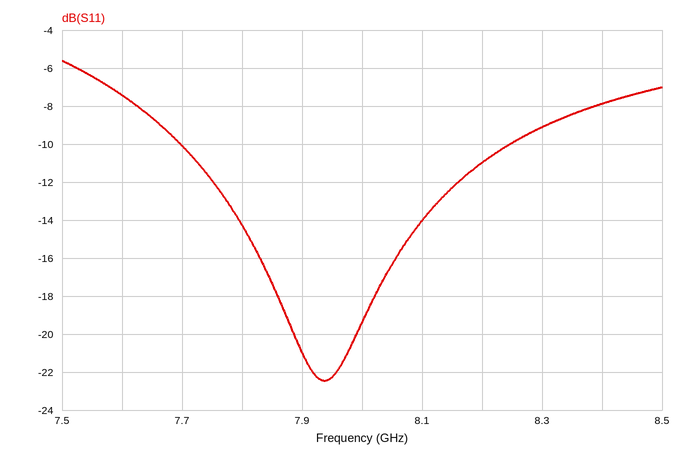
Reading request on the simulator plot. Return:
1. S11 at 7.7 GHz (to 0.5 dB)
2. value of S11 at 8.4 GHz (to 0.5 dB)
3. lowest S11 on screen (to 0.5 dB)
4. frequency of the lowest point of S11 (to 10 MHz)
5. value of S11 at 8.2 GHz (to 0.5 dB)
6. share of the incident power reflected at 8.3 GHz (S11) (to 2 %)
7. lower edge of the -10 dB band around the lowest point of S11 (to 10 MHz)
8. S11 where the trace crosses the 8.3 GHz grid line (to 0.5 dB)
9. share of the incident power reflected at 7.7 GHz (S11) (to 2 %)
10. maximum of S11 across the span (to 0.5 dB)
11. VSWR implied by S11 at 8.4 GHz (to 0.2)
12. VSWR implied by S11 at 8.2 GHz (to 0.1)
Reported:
-10.0 dB
-8.0 dB
-22.5 dB
7.94 GHz
-11.0 dB
12 %
7.70 GHz
-9.0 dB
10 %
-5.5 dB
2.4
1.8
